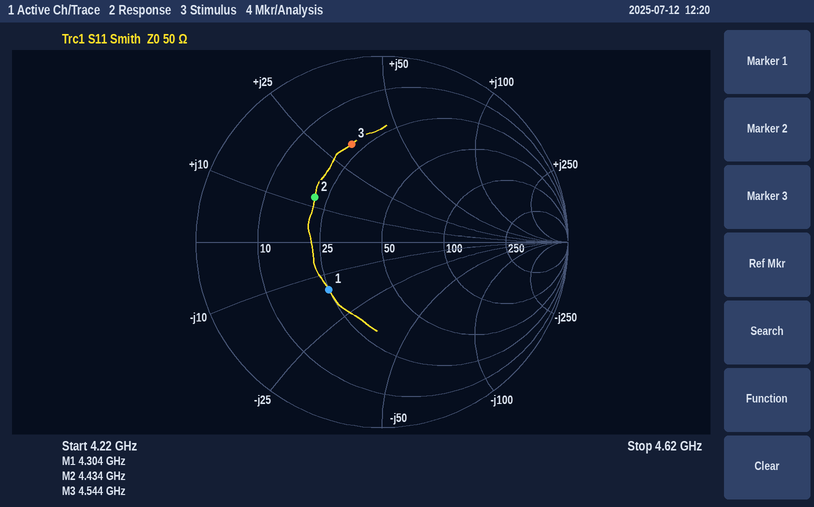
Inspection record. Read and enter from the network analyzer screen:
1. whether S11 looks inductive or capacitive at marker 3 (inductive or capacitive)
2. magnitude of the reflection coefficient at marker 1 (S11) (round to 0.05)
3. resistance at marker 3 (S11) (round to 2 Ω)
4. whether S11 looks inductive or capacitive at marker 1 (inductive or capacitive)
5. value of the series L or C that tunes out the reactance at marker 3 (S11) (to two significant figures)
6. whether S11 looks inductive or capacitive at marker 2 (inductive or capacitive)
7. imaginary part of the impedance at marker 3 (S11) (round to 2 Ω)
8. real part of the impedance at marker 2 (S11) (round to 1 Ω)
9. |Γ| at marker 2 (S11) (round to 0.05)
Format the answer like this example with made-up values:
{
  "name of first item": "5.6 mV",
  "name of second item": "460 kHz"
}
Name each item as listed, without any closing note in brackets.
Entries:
{
  "whether S11 looks inductive or capacitive at marker 3": "inductive",
  "magnitude of the reflection coefficient at marker 1 (S11)": "0.40",
  "resistance at marker 3 (S11)": "22 Ω",
  "whether S11 looks inductive or capacitive at marker 1": "capacitive",
  "value of the series L or C that tunes out the reactance at marker 3 (S11)": "1.1 pF",
  "whether S11 looks inductive or capacitive at marker 2": "inductive",
  "imaginary part of the impedance at marker 3 (S11)": "+32 Ω",
  "real part of the impedance at marker 2 (S11)": "21 Ω",
  "|Γ| at marker 2 (S11)": "0.45"
}
